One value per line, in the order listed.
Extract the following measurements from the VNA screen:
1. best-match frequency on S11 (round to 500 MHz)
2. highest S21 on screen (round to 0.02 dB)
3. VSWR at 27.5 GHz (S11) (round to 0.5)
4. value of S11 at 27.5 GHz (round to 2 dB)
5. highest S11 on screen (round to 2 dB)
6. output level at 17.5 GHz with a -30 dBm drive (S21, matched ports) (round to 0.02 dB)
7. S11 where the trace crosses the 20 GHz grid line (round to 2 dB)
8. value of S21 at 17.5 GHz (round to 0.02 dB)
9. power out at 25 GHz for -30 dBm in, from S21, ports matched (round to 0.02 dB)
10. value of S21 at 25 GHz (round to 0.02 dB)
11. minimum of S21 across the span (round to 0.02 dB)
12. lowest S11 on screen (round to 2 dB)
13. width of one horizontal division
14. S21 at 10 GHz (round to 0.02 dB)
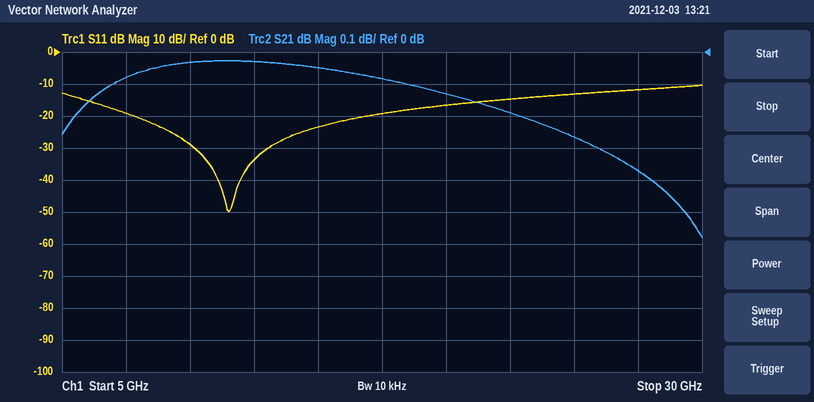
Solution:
11.5 GHz
-0.02 dB
1.5
-12 dB
-10 dB
-30.08 dBm
-16 dB
-0.08 dB
-30.26 dBm
-0.26 dB
-0.58 dB
-50 dB
2.5 GHz
-0.04 dB
